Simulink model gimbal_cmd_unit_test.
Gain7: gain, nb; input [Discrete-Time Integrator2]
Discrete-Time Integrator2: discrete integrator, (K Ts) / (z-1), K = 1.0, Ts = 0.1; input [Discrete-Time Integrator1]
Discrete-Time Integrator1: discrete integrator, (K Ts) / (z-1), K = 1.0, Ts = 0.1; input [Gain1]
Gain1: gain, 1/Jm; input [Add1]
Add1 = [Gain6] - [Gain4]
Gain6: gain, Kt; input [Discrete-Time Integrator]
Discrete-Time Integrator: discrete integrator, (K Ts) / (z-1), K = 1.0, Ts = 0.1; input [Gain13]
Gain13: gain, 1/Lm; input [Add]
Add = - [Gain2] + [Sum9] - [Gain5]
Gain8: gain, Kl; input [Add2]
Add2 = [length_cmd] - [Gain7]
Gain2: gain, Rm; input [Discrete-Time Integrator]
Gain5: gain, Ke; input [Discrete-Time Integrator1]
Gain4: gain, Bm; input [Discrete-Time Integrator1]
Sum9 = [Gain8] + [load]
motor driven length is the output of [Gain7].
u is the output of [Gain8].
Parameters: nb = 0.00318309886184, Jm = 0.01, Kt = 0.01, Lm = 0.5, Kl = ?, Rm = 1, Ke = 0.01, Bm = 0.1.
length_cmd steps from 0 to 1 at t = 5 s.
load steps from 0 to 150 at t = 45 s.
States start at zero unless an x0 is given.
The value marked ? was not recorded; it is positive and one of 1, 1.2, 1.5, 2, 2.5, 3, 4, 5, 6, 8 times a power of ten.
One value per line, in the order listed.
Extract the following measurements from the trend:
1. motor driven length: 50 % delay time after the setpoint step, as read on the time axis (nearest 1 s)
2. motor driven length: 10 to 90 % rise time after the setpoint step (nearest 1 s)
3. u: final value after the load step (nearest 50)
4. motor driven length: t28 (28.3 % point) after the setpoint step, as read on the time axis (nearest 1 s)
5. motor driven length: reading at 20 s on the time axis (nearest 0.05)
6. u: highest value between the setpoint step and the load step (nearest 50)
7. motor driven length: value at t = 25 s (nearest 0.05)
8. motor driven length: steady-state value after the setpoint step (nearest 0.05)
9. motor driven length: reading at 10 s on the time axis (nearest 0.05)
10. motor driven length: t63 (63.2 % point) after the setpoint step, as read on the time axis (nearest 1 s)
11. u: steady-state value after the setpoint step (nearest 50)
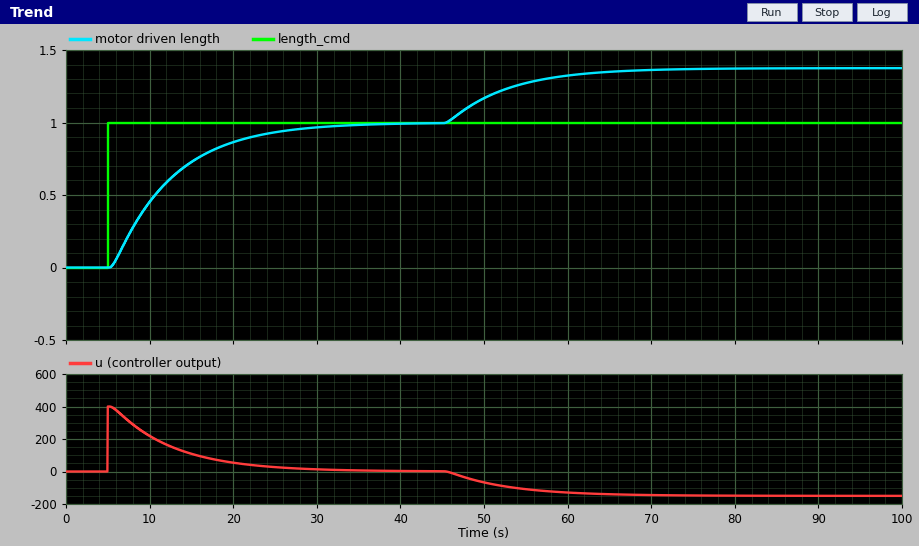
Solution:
11 s
16 s
-150
8 s
0.85
400
0.95
1.00
0.45
13 s
0
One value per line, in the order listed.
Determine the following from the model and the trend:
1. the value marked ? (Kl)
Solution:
400
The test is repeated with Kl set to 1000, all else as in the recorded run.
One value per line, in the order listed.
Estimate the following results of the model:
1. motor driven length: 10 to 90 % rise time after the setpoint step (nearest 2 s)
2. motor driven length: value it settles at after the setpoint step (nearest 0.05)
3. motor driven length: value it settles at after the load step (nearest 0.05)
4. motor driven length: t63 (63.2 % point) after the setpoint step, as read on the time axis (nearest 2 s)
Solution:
6 s
1.00
1.15
8 s
